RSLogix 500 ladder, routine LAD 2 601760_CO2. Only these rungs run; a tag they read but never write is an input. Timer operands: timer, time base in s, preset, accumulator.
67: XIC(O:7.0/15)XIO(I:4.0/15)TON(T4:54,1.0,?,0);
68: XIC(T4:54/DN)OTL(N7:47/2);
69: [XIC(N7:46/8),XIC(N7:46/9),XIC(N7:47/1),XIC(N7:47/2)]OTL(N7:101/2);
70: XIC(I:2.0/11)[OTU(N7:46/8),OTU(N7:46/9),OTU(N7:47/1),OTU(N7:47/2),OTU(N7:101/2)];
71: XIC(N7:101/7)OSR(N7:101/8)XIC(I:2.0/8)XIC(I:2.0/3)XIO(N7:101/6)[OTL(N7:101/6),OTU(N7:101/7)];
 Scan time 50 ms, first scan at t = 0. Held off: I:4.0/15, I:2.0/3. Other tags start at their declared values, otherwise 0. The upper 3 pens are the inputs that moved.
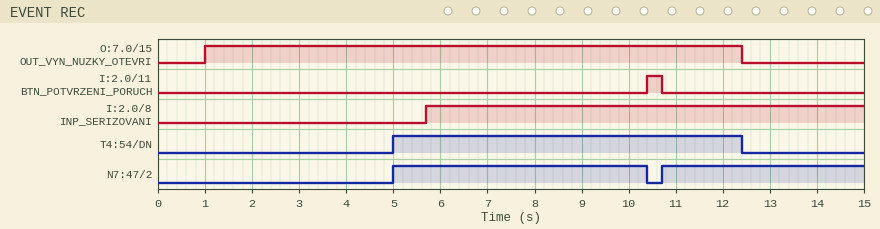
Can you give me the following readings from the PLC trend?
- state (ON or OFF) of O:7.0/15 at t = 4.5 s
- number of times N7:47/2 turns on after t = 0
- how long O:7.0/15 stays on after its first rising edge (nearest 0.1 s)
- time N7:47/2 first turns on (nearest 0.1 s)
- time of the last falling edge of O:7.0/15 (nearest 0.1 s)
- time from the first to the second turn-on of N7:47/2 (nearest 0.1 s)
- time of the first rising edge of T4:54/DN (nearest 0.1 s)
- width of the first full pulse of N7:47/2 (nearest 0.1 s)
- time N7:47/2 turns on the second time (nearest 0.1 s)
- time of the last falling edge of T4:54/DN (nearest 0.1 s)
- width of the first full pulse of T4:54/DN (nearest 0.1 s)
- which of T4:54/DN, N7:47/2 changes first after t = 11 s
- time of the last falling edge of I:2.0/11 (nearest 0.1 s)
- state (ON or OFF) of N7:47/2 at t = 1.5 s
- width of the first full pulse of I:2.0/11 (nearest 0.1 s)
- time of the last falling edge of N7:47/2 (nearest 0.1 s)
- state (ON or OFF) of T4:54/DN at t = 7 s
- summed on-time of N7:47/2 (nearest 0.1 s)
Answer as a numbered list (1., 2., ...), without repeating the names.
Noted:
1. ON
2. 2
3. 11.4 s
4. 5.0 s
5. 12.4 s
6. 5.7 s
7. 5.0 s
8. 5.4 s
9. 10.7 s
10. 12.4 s
11. 7.4 s
12. T4:54/DN
13. 10.7 s
14. OFF
15. 0.3 s
16. 10.4 s
17. ON
18. 9.7 s
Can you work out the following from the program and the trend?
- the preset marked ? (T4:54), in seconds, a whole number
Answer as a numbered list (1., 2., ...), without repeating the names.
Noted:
1. 4 s
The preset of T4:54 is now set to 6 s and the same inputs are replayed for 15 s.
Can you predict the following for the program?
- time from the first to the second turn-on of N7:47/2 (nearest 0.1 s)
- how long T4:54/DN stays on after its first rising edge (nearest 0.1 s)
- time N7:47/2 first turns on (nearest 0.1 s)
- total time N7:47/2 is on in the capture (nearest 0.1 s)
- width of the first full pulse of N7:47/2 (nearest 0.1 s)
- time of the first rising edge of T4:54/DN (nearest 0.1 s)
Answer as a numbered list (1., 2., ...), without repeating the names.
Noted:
1. 3.7 s
2. 5.4 s
3. 7.0 s
4. 7.7 s
5. 3.4 s
6. 7.0 s
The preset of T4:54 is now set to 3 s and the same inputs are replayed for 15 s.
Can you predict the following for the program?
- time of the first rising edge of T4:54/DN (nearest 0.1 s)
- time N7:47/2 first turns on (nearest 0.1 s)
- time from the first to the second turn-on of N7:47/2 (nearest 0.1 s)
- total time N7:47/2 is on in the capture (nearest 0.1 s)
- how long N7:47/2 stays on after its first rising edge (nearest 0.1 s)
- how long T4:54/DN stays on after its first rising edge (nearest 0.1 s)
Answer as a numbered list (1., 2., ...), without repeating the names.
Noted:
1. 4.0 s
2. 4.0 s
3. 6.7 s
4. 10.7 s
5. 6.4 s
6. 8.4 s
